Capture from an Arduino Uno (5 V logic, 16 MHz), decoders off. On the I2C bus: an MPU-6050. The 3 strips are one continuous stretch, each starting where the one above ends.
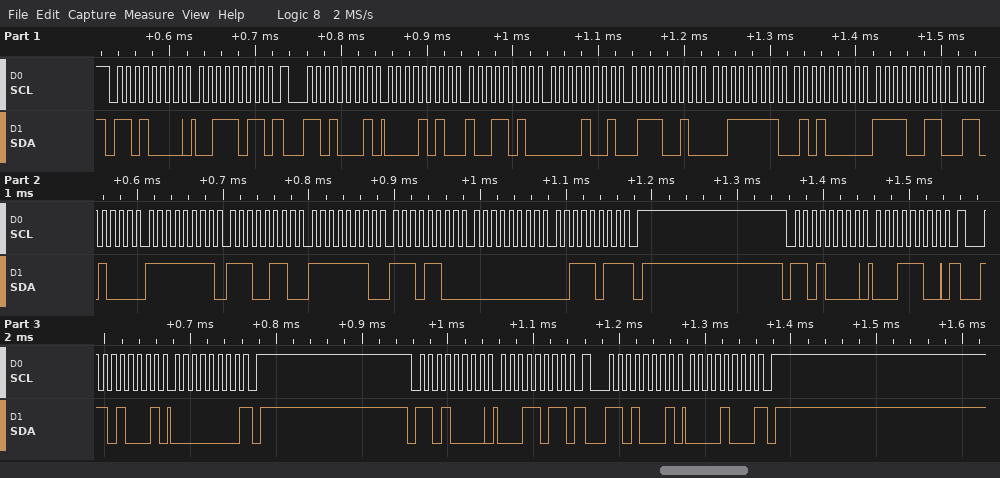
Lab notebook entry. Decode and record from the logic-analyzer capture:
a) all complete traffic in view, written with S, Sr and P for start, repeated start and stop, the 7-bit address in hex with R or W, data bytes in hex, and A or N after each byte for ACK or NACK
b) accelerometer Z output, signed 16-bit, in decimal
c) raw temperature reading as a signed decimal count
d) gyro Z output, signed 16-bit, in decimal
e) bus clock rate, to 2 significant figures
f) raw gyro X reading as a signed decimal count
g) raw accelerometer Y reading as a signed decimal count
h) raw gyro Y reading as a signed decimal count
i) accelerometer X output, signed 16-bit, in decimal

S 68W A 3B A Sr 68R A 0A A 9A A 09 A 72 A 3F A 50 A F3 A 68 A FF A E6 A FE A EC A 00 A 3B N P S 68W A 1C A Sr 68R A 00 N P S 68W A 1B A Sr 68R A 08 N P
16208
-3224
59
100 kHz
-26
2418
-276
2714
